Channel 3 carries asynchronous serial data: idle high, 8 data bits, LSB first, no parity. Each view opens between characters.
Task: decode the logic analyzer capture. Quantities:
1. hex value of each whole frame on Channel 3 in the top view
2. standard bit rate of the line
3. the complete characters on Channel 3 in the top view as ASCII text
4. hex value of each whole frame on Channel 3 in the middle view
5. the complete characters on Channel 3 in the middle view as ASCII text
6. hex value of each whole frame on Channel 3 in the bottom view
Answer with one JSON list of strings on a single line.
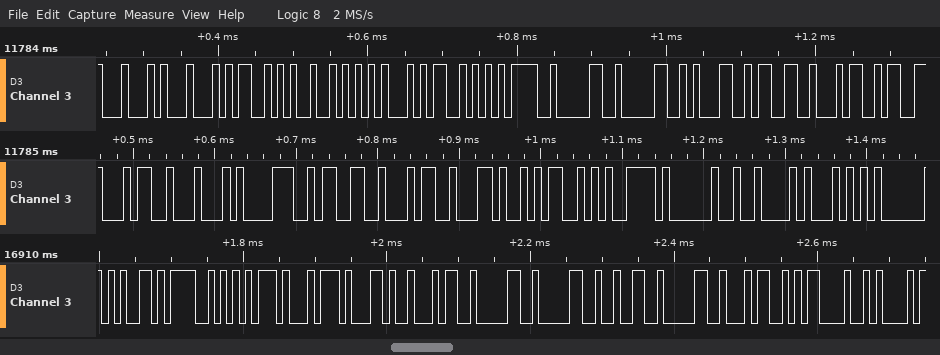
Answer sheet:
["44, 44, 53, 52, 45, 53, 3D, 30, 30, 31, 33, 34", "115200 baud", "\"DDSRES=00134\"", "34, 44, 38, 33, 34, 2C, 4D, 79, 20, 42, 54", "\"4D834,My BT\"", "65, 4F, 75, 74, 2C, 34, 30, 30, 32, 30, 34, 0D, 0A"]
